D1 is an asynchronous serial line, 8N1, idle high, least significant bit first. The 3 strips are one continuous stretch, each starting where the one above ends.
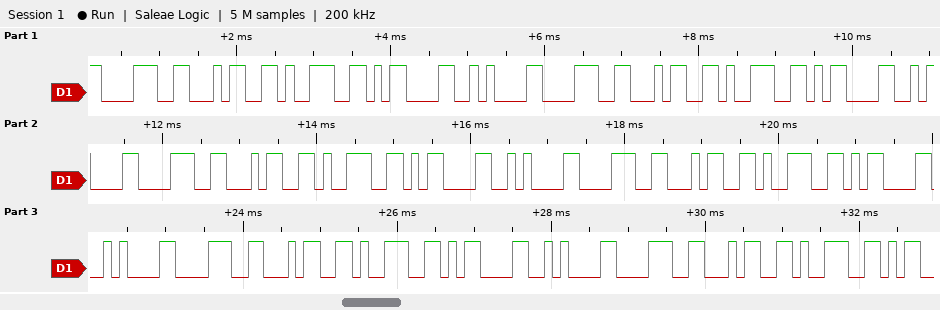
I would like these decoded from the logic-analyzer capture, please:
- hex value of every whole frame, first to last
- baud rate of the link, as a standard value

38 34 39 0D 0A 38 34 39 0D 0A 38 34 39 0D 0A 38 34 39 0D 0A 38 34 39 0D 0A 38 34 39
9600 baud
